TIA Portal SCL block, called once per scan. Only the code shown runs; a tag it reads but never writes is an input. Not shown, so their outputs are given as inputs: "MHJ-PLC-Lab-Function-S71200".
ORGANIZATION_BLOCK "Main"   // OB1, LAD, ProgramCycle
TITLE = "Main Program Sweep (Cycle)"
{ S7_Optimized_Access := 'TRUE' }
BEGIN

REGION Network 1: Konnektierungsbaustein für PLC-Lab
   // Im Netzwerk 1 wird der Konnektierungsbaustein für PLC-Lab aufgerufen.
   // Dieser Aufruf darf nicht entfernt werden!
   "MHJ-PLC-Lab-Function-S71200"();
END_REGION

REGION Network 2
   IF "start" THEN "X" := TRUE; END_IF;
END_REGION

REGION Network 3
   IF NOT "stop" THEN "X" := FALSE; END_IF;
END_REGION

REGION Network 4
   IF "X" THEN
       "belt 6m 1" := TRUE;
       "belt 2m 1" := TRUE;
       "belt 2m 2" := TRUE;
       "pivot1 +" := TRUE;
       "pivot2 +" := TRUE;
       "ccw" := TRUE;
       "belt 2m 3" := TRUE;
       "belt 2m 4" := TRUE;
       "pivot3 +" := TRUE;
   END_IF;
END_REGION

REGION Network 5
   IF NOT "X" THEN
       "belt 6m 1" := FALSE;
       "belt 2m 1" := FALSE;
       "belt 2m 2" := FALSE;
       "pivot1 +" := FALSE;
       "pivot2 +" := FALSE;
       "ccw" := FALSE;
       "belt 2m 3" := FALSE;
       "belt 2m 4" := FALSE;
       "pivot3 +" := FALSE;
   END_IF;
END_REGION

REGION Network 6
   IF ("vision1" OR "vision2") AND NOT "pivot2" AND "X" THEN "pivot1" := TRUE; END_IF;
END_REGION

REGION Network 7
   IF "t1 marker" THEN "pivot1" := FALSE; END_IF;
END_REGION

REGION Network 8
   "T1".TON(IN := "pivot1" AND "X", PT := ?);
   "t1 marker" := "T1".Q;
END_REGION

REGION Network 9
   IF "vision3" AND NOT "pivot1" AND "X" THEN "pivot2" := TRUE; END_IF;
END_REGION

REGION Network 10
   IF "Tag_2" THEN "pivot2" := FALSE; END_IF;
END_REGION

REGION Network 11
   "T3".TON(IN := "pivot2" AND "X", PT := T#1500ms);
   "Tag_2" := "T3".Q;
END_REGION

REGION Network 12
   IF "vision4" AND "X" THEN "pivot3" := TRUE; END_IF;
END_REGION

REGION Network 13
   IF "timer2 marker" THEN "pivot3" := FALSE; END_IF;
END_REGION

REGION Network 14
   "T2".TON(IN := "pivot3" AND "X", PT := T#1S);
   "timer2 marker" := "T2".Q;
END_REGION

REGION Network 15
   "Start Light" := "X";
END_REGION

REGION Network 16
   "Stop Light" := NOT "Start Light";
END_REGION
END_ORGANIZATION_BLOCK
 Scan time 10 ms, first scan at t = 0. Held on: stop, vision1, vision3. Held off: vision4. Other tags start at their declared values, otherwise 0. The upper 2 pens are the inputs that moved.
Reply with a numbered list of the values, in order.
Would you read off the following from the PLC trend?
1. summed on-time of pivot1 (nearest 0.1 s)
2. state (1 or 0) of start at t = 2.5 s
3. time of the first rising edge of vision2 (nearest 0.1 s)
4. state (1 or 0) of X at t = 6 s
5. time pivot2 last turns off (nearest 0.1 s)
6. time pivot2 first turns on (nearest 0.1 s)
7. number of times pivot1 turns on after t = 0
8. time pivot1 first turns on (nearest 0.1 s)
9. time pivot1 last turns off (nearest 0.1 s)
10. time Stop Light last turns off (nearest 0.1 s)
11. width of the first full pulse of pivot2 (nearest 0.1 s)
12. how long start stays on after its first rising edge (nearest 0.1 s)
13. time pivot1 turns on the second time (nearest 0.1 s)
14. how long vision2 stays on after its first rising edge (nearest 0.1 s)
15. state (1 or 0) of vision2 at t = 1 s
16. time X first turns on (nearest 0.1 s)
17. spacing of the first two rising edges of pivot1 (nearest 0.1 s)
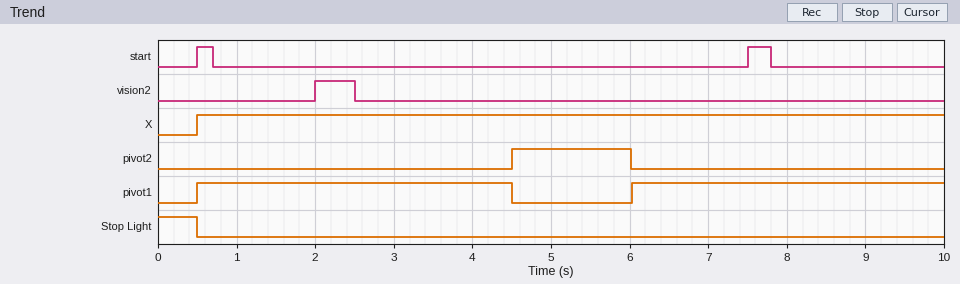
1. 8.0 s
2. 0
3. 2.0 s
4. 1
5. 6.0 s
6. 4.5 s
7. 2
8. 0.5 s
9. 4.5 s
10. 0.5 s
11. 1.5 s
12. 0.2 s
13. 6.0 s
14. 0.5 s
15. 0
16. 0.5 s
17. 5.5 s
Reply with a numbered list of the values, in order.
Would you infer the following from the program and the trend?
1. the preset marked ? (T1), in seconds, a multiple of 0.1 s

1. 4.0 s
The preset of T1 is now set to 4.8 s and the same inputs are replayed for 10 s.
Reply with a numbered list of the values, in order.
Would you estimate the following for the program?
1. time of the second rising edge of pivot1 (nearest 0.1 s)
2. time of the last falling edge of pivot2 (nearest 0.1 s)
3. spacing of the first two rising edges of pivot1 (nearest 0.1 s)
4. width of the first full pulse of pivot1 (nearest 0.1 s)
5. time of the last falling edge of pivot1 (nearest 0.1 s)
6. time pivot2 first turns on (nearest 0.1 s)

1. 6.8 s
2. 6.8 s
3. 6.3 s
4. 4.8 s
5. 5.3 s
6. 5.3 s
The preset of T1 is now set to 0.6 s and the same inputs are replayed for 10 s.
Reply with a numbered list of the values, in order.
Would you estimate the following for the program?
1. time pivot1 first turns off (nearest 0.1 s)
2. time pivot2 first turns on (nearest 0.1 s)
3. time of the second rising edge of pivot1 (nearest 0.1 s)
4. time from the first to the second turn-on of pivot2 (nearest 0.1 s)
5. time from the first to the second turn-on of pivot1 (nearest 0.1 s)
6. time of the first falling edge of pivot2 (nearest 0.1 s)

1. 1.1 s
2. 1.1 s
3. 2.6 s
4. 2.1 s
5. 2.1 s
6. 2.6 s
